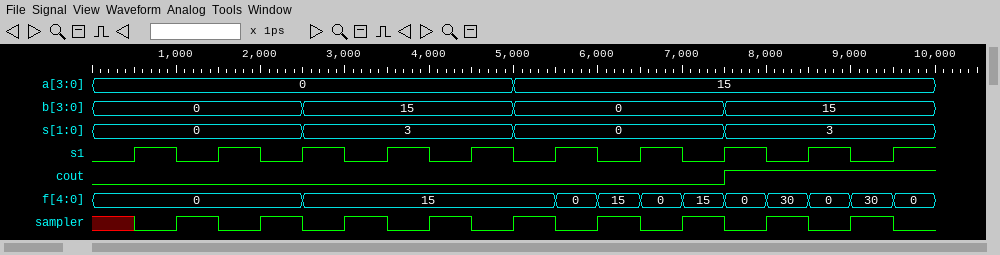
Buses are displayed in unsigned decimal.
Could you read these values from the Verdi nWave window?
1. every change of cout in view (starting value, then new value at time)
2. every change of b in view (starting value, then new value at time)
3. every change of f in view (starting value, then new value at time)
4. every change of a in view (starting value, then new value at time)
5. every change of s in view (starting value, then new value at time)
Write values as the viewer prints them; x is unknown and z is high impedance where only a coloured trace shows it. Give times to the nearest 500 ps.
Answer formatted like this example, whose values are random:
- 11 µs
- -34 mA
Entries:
- 0, 1 at 7500 ps
- 0, 15 at 2500 ps, 0 at 5000 ps, 15 at 7500 ps
- 0, 15 at 2500 ps, 0 at 5500 ps, 15 at 6000 ps, 0 at 6500 ps, 15 at 7000 ps, 0 at 7500 ps, 30 at 8000 ps, 0 at 8500 ps, 30 at 9000 ps, 0 at 9500 ps
- 0, 15 at 5000 ps
- 0, 3 at 2500 ps, 0 at 5000 ps, 3 at 7500 ps
